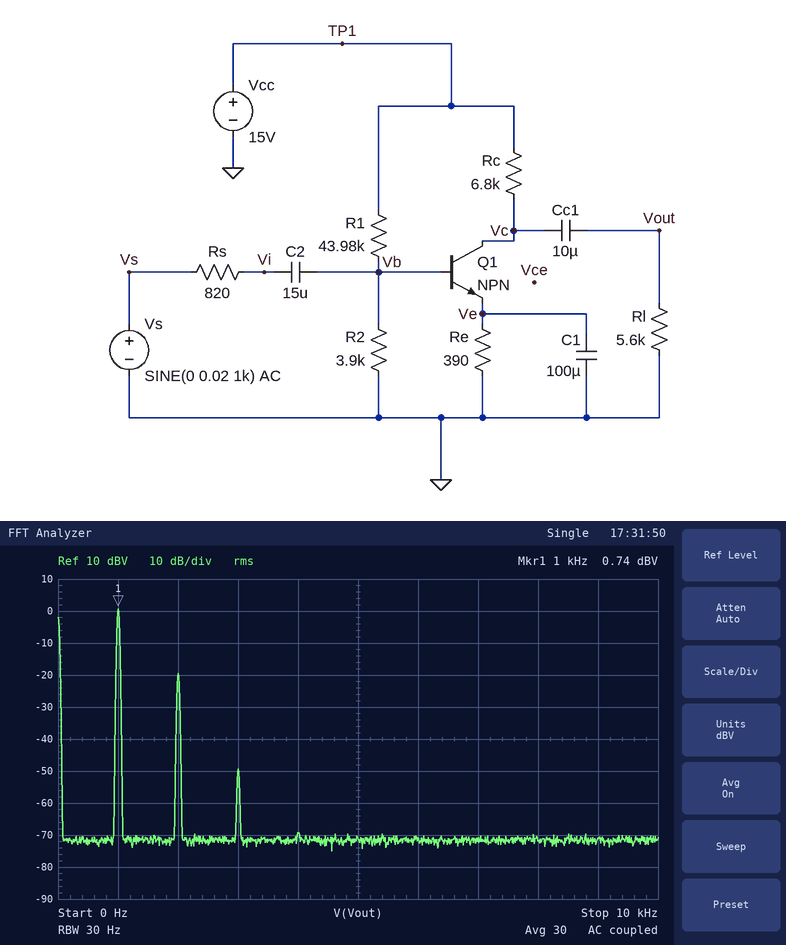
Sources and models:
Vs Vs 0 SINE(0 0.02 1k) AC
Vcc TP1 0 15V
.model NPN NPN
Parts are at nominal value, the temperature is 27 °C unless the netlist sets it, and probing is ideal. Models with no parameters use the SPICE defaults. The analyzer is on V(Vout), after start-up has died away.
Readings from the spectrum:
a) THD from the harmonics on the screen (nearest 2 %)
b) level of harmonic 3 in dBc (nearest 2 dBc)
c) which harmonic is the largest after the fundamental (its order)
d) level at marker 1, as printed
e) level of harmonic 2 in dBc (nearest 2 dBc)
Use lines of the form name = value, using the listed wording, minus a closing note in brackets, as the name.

THD from the harmonics on the screen = 10 %
level of harmonic 3 in dBc = -50 dBc
which harmonic is the largest after the fundamental = 2
level at marker 1, as printed = 0.74 dBV
level of harmonic 2 in dBc = -20 dBc
